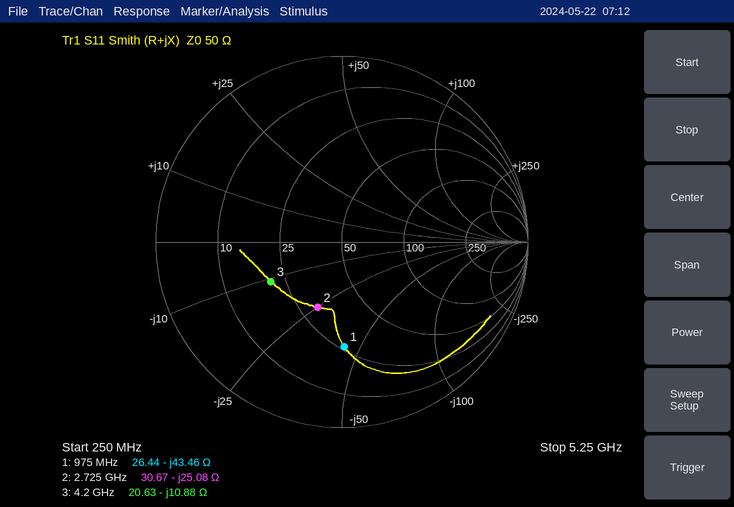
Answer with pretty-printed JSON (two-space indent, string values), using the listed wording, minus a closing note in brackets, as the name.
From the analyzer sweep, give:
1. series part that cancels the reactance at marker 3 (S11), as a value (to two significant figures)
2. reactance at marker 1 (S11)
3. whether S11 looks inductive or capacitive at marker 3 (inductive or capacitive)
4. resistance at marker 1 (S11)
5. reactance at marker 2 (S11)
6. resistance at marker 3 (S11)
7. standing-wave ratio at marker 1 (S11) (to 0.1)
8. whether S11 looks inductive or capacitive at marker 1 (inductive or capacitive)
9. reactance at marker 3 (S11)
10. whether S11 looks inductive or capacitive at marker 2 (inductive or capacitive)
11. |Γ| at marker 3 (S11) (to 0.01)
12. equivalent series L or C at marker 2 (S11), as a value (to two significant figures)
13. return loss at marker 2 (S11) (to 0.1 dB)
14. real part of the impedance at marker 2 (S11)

{
  "series part that cancels the reactance at marker 3 (S11), as a value": "410 pH",
  "reactance at marker 1": "-43.46 Ω",
  "whether S11 looks inductive or capacitive at marker 3": "capacitive",
  "resistance at marker 1": "26.44 Ω",
  "reactance at marker 2": "-25.08 Ω",
  "resistance at marker 3": "20.63 Ω",
  "standing-wave ratio at marker 1 (S11)": "3.6",
  "whether S11 looks inductive or capacitive at marker 1": "capacitive",
  "reactance at marker 3": "-10.88 Ω",
  "whether S11 looks inductive or capacitive at marker 2": "capacitive",
  "|Γ| at marker 3 (S11)": "0.44",
  "equivalent series L or C at marker 2 (S11), as a value": "2.3 pF",
  "return loss at marker 2 (S11)": "8.5 dB",
  "real part of the impedance at marker 2": "30.67 Ω"
}
